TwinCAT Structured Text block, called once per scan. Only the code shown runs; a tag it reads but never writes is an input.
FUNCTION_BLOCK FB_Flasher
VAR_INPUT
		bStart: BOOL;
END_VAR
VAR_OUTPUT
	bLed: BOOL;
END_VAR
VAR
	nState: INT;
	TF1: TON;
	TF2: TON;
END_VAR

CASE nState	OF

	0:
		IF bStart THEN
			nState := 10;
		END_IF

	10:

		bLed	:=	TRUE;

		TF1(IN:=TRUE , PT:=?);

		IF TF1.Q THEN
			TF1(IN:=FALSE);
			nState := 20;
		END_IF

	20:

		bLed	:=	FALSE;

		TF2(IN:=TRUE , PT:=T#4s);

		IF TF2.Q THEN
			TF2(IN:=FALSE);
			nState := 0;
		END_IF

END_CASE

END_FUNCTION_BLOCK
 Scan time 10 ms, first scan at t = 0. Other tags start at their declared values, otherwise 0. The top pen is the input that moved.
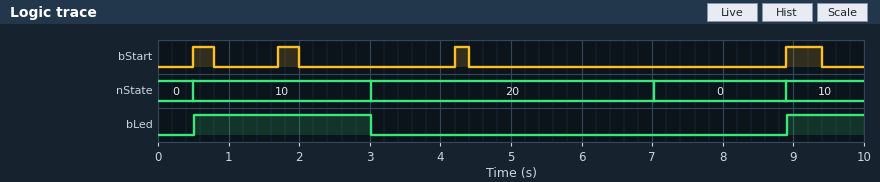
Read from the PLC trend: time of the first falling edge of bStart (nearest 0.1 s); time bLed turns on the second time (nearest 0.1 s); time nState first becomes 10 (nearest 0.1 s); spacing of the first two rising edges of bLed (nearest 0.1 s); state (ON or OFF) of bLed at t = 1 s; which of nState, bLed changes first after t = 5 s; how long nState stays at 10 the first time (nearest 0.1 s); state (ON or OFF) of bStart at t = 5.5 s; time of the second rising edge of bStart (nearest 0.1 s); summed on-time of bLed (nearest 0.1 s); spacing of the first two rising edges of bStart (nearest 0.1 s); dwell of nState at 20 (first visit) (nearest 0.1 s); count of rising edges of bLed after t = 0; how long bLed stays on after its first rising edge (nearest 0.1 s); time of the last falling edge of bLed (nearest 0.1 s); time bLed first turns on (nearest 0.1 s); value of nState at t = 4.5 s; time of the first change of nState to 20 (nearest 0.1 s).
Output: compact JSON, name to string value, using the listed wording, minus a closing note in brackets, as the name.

{"time of the first falling edge of bStart": "0.8 s", "time bLed turns on the second time": "8.9 s", "time nState first becomes 10": "0.5 s", "spacing of the first two rising edges of bLed": "8.4 s", "state (ON or OFF) of bLed at t = 1 s": "ON", "which of nState, bLed changes first after t = 5 s": "nState", "how long nState stays at 10 the first time": "2.5 s", "state (ON or OFF) of bStart at t = 5.5 s": "OFF", "time of the second rising edge of bStart": "1.7 s", "summed on-time of bLed": "3.6 s", "spacing of the first two rising edges of bStart": "1.2 s", "dwell of nState at 20 (first visit)": "4.0 s", "count of rising edges of bLed after t = 0": "2", "how long bLed stays on after its first rising edge": "2.5 s", "time of the last falling edge of bLed": "3.0 s", "time bLed first turns on": "0.5 s", "value of nState at t = 4.5 s": "20", "time of the first change of nState to 20": "3.0 s"}
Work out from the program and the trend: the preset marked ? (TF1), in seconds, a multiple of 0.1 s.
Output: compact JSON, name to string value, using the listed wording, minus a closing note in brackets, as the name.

{"the preset marked ? (TF1), in seconds, a multiple of 0.1 s": "2.5 s"}
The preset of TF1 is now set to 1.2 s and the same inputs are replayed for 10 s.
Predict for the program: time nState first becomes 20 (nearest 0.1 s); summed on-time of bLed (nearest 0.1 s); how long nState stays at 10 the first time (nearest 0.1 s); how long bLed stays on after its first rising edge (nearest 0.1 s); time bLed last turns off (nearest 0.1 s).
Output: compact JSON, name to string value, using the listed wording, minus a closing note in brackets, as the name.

{"time nState first becomes 20": "1.7 s", "summed on-time of bLed": "2.3 s", "how long nState stays at 10 the first time": "1.2 s", "how long bLed stays on after its first rising edge": "1.2 s", "time bLed last turns off": "1.7 s"}
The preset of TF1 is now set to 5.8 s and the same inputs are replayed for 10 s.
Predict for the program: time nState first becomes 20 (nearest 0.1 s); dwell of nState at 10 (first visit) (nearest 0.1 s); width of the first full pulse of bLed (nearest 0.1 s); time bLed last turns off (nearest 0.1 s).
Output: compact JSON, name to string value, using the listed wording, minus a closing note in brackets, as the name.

{"time nState first becomes 20": "6.3 s", "dwell of nState at 10 (first visit)": "5.8 s", "width of the first full pulse of bLed": "5.8 s", "time bLed last turns off": "6.3 s"}
